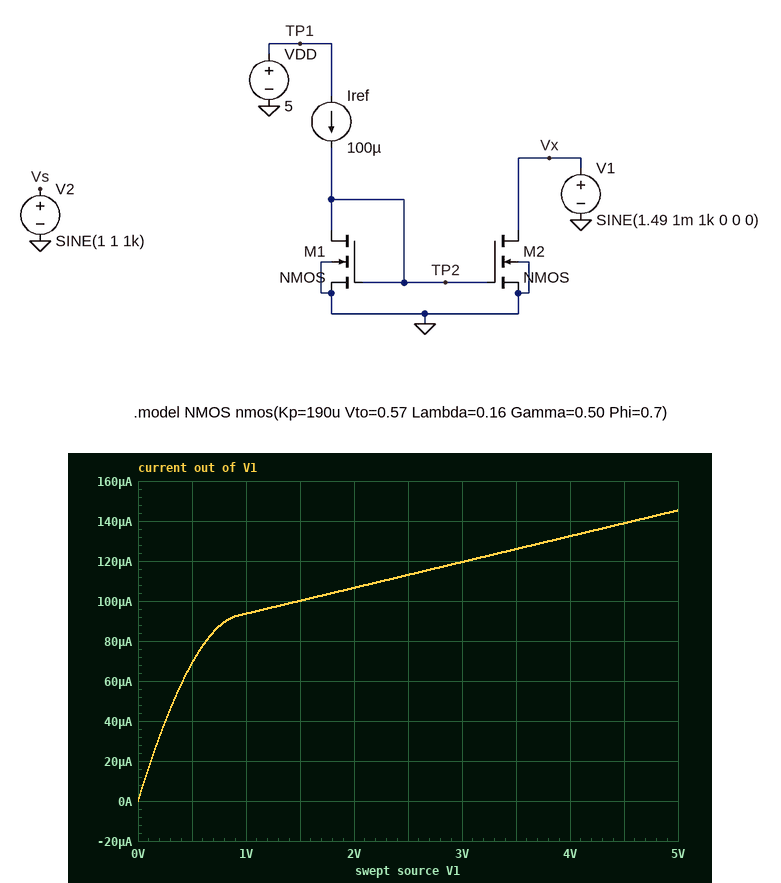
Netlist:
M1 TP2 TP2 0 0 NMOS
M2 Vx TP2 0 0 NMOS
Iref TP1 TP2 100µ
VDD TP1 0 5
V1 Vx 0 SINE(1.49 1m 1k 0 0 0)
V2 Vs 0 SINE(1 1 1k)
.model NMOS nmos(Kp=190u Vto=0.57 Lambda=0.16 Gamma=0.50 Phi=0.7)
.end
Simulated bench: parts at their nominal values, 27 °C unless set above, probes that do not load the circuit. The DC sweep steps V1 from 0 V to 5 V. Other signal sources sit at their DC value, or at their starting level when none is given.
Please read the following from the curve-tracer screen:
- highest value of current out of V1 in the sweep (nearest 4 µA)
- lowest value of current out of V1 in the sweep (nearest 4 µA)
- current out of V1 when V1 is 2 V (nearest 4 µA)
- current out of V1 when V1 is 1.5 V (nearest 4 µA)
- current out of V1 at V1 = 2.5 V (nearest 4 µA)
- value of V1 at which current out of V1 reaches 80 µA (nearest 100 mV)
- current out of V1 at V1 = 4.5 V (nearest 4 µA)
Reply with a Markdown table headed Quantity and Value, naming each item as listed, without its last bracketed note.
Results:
| Quantity | Value |
|---|---|
| highest value of current out of V1 in the sweep | 144 µA |
| lowest value of current out of V1 in the sweep | 0 A |
| current out of V1 when V1 is 2 V | 108 µA |
| current out of V1 when V1 is 1.5 V | 100 µA |
| current out of V1 at V1 = 2.5 V | 112 µA |
| value of V1 at which current out of V1 reaches 80 µA | 600 mV |
| current out of V1 at V1 = 4.5 V | 140 µA |
